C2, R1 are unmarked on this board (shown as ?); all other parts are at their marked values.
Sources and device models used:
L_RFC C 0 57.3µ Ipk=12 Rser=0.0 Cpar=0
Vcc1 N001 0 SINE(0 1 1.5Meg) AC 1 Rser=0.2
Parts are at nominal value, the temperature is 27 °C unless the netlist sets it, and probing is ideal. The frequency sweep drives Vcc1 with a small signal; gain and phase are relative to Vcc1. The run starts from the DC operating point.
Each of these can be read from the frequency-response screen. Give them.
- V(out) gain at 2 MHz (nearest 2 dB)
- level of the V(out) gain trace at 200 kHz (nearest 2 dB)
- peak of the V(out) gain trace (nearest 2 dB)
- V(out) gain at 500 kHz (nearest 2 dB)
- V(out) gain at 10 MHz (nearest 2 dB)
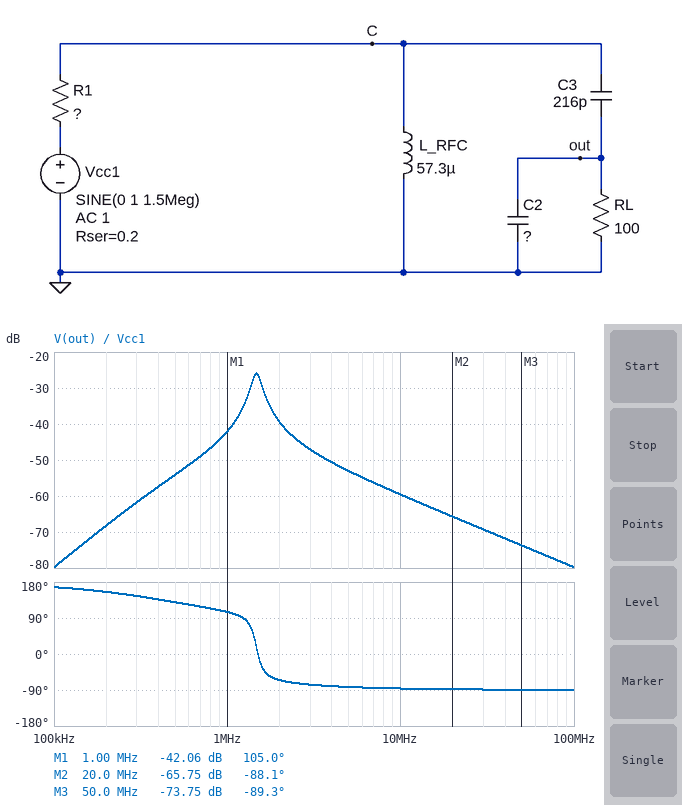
-40 dB
-68 dB
-26 dB
-54 dB
-60 dB
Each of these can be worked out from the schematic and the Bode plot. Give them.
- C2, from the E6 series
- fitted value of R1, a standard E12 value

3.3 nF
4.7 kΩ
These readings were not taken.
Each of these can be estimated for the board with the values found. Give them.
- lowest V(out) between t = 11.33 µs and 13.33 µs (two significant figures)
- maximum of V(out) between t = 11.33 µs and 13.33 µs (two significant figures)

-49 mV
49 mV
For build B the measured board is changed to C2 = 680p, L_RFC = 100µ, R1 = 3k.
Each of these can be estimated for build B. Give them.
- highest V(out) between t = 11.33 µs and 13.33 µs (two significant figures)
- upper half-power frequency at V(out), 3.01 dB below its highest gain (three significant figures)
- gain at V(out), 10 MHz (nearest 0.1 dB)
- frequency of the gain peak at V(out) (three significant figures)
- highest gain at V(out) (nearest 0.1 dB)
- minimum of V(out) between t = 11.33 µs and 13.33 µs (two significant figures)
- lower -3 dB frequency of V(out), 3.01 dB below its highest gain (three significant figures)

54 mV
1.41 MHz
-42.3 dB
1.13 MHz
-21.3 dB
-54 mV
961 kHz
